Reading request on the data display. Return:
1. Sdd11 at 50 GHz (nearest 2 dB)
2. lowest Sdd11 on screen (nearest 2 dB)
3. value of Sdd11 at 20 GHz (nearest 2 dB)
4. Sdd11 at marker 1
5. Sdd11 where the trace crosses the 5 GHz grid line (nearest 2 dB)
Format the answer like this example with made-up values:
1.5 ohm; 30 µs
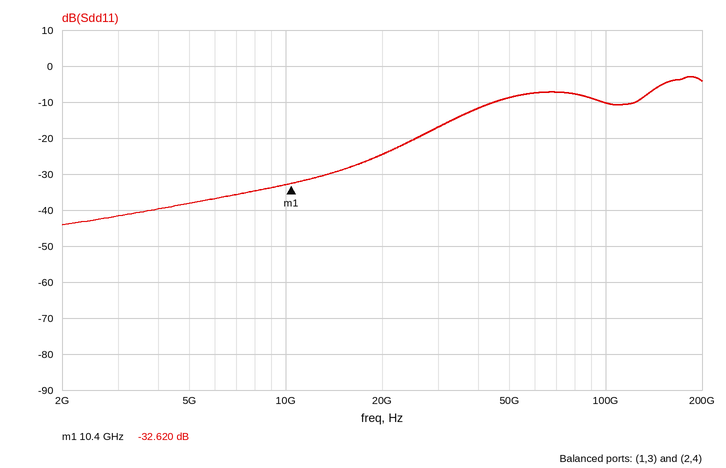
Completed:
-8 dB; -44 dB; -24 dB; -32.620 dB; -38 dB
